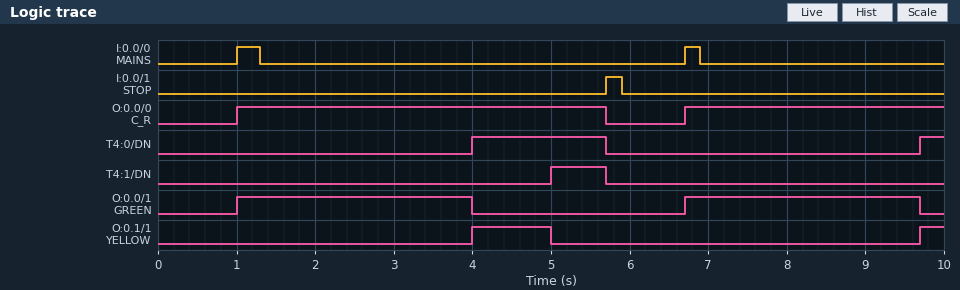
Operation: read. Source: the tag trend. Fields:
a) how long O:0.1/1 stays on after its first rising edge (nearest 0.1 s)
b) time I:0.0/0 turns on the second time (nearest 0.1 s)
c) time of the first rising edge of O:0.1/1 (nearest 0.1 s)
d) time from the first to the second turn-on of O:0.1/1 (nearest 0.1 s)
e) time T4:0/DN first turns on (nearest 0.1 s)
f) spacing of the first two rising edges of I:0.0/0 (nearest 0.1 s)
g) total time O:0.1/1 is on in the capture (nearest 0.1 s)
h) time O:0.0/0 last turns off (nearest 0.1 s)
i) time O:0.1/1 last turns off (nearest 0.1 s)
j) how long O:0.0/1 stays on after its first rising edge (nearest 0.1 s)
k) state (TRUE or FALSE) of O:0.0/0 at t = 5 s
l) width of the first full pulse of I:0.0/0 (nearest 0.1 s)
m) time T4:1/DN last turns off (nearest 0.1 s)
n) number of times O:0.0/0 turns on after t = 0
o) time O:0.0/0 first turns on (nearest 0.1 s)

1.0 s
6.7 s
4.0 s
5.7 s
4.0 s
5.7 s
1.3 s
5.7 s
5.0 s
3.0 s
TRUE
0.3 s
5.7 s
2
1.0 s
